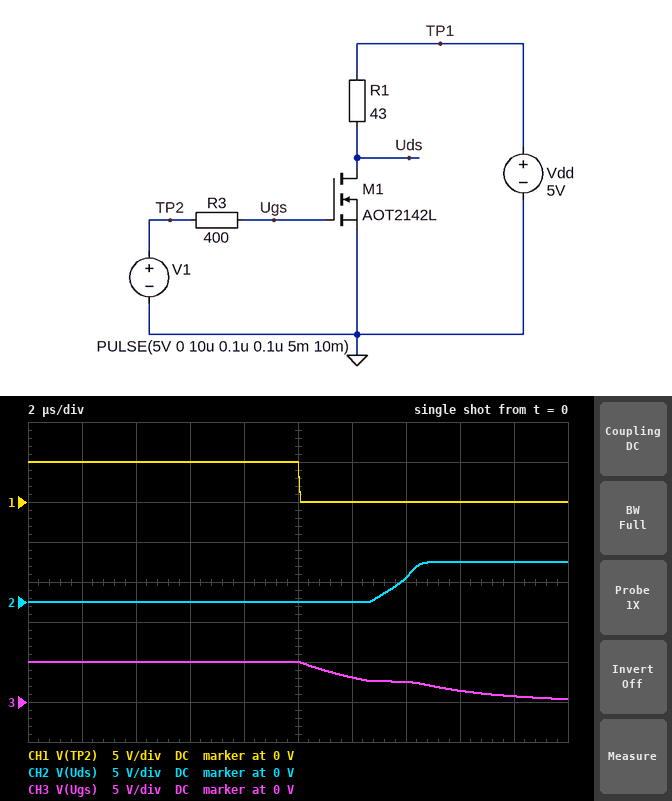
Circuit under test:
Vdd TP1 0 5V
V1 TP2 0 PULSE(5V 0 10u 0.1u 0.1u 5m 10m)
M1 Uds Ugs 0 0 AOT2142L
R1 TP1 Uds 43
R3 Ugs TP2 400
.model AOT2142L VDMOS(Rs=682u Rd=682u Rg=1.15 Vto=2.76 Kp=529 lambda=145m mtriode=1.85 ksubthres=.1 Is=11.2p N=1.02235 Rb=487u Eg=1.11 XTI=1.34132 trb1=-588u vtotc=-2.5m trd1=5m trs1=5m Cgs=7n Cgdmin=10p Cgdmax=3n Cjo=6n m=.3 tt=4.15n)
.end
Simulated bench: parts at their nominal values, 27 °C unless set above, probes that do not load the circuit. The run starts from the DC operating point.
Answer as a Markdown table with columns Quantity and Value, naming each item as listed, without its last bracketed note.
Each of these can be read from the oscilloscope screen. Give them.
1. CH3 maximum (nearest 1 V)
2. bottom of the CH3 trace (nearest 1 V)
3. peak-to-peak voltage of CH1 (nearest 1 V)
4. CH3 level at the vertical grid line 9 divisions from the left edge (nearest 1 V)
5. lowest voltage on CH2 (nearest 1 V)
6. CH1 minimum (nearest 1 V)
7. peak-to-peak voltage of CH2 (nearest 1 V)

| Quantity | Value |
|---|---|
| CH3 maximum | 5 V |
| bottom of the CH3 trace | 0 V |
| peak-to-peak voltage of CH1 | 5 V |
| CH3 level at the vertical grid line 9 divisions from the left edge | 1 V |
| lowest voltage on CH2 | 0 V |
| CH1 minimum | 0 V |
| peak-to-peak voltage of CH2 | 5 V |
